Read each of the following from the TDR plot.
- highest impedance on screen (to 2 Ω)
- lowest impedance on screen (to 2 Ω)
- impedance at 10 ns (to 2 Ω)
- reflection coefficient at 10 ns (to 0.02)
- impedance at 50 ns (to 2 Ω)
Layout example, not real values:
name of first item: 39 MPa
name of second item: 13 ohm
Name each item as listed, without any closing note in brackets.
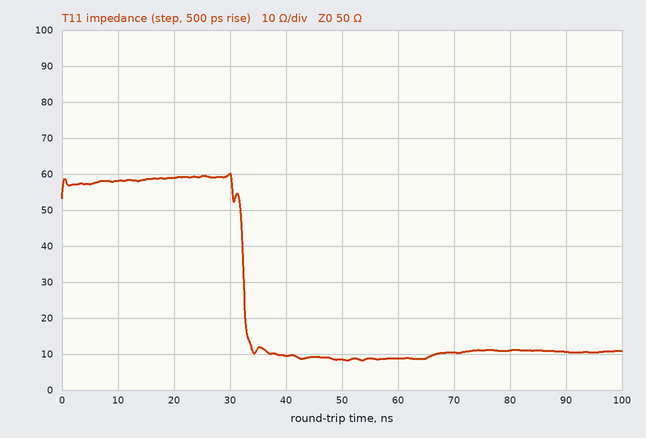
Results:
highest impedance on screen: 60 Ω
lowest impedance on screen: 8 Ω
impedance at 10 ns: 58 Ω
reflection coefficient at 10 ns: +0.08
impedance at 50 ns: 8 Ω
